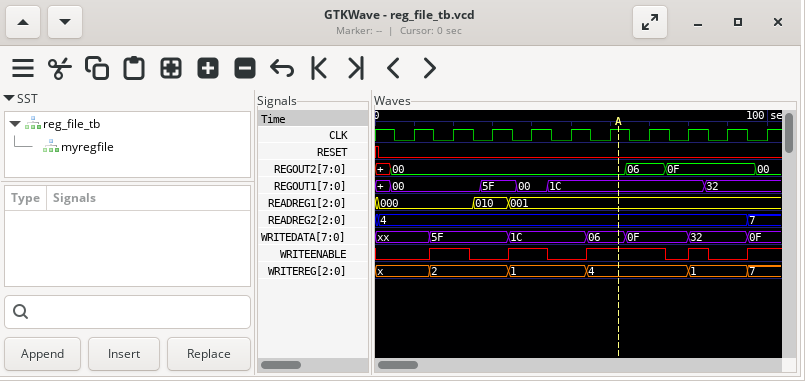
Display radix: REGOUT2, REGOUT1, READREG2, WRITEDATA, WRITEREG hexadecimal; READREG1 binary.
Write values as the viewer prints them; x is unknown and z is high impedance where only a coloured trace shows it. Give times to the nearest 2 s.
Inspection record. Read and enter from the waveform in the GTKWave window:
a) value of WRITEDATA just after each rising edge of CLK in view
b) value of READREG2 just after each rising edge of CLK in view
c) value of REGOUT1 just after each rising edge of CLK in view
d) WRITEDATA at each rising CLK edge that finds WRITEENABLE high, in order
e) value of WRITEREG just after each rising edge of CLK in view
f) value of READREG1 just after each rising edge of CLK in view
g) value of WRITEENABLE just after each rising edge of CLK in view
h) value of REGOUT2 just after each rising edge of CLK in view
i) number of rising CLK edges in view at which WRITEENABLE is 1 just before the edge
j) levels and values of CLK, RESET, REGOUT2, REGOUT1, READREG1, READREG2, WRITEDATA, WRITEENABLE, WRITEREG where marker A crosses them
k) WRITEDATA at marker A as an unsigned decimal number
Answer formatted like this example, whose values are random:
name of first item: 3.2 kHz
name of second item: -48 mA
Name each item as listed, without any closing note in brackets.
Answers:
value of WRITEDATA just after each rising edge of CLK in view: xx, 5F, 5F, 1C, 1C, 06, 0F, 32, 32, 0F
value of READREG2 just after each rising edge of CLK in view: 4, 4, 4, 4, 4, 4, 4, 4, 4, 7
value of REGOUT1 just after each rising edge of CLK in view: 00, 00, 5F, 00, 1C, 1C, 1C, 1C, 32, 32
WRITEDATA at each rising CLK edge that finds WRITEENABLE high, in order: 5F, 1C, 06, 0F, 0F
value of WRITEREG just after each rising edge of CLK in view: x, 2, 2, 1, 1, 4, 4, 1, 1, 7
value of READREG1 just after each rising edge of CLK in view: 000, 000, 010, 001, 001, 001, 001, 001, 001, 001
value of WRITEENABLE just after each rising edge of CLK in view: 0 1 0 1 0 1 1 1 0 1
value of REGOUT2 just after each rising edge of CLK in view: 00, 00, 00, 00, 00, 00, 06, 0F, 0F, 00
number of rising CLK edges in view at which WRITEENABLE is 1 just before the edge: 5
levels and values of CLK, RESET, REGOUT2, REGOUT1, READREG1, READREG2, WRITEDATA, WRITEENABLE, WRITEREG where marker A crosses them: CLK=1, RESET=0, REGOUT2=00, REGOUT1=1C, READREG1=001, READREG2=4, WRITEDATA=06, WRITEENABLE=1, WRITEREG=4
WRITEDATA at marker A as an unsigned decimal number: 6
